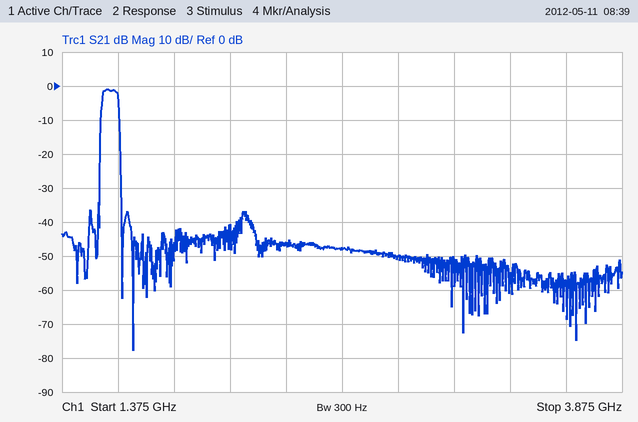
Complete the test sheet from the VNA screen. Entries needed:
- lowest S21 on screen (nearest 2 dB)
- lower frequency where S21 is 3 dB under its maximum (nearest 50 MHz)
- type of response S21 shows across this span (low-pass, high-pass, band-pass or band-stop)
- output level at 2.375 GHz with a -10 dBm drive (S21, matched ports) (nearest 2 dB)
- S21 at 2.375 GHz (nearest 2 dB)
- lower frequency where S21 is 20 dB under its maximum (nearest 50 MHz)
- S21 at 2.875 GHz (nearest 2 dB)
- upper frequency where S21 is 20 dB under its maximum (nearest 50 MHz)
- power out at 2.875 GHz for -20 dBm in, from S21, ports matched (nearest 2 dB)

-78 dB
1.55 GHz
band-pass
-56 dBm
-46 dB
1.55 GHz
-50 dB
1.65 GHz
-70 dBm
